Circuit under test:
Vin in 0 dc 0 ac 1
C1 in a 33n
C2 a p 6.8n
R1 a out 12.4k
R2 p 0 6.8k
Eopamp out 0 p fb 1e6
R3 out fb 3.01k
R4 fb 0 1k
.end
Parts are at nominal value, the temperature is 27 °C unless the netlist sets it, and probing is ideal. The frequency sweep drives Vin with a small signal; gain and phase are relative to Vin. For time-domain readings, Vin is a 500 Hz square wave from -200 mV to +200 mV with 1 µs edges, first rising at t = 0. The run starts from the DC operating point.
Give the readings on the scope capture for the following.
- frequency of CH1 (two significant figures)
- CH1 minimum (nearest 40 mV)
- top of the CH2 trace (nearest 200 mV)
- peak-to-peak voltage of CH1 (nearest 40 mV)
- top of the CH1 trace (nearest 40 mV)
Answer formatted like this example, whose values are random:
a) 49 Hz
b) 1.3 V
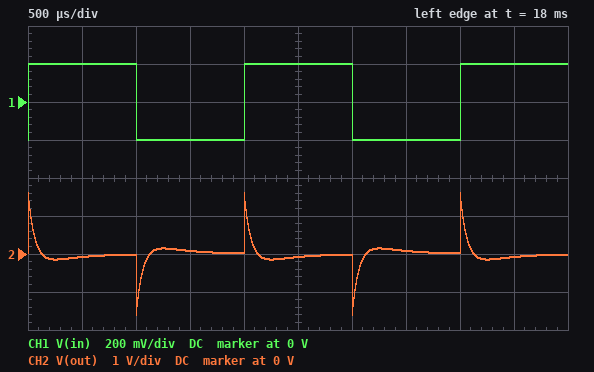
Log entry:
a) 500 Hz
b) -200 mV
c) 1.6 V
d) 400 mV
e) 200 mV
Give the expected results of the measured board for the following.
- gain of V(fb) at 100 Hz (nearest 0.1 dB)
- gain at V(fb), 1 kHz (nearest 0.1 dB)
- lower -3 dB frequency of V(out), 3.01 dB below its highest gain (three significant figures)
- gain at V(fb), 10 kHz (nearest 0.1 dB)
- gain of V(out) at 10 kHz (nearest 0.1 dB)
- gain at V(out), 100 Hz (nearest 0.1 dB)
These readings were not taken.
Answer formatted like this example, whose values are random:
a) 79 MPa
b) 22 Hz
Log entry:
a) -42.7 dB
b) -9.5 dB
c) 2.55 kHz
d) -0.3 dB
e) 11.8 dB
f) -30.6 dB
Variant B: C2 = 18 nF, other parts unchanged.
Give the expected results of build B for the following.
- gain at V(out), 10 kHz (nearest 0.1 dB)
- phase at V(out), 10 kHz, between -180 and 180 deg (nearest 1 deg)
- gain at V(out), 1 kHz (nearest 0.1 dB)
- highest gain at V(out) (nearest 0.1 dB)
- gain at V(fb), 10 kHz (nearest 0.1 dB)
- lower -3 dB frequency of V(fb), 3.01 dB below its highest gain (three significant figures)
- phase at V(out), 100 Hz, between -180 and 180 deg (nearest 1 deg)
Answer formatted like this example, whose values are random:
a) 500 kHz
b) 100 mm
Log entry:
a) 12.1 dB
b) 5 deg
c) 12.3 dB
d) 12.5 dB
e) 0 dB
f) 634 Hz
g) 170 deg
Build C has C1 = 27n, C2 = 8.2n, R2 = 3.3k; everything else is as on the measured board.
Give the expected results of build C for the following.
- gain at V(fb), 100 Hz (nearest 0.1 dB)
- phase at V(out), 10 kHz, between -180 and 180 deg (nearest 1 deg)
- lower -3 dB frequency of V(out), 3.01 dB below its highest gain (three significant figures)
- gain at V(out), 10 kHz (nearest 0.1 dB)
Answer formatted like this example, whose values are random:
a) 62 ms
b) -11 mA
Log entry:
a) -49.1 dB
b) 33 deg
c) 5.79 kHz
d) 10.8 dB
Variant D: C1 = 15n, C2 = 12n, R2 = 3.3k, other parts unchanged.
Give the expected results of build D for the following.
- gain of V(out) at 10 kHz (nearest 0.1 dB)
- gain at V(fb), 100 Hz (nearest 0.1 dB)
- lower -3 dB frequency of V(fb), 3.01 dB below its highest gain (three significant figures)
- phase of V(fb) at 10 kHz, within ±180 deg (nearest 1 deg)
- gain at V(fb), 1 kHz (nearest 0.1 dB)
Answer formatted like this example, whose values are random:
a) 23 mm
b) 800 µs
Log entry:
a) 11.5 dB
b) -50.8 dB
c) 3.95 kHz
d) 26 deg
e) -14.4 dB
